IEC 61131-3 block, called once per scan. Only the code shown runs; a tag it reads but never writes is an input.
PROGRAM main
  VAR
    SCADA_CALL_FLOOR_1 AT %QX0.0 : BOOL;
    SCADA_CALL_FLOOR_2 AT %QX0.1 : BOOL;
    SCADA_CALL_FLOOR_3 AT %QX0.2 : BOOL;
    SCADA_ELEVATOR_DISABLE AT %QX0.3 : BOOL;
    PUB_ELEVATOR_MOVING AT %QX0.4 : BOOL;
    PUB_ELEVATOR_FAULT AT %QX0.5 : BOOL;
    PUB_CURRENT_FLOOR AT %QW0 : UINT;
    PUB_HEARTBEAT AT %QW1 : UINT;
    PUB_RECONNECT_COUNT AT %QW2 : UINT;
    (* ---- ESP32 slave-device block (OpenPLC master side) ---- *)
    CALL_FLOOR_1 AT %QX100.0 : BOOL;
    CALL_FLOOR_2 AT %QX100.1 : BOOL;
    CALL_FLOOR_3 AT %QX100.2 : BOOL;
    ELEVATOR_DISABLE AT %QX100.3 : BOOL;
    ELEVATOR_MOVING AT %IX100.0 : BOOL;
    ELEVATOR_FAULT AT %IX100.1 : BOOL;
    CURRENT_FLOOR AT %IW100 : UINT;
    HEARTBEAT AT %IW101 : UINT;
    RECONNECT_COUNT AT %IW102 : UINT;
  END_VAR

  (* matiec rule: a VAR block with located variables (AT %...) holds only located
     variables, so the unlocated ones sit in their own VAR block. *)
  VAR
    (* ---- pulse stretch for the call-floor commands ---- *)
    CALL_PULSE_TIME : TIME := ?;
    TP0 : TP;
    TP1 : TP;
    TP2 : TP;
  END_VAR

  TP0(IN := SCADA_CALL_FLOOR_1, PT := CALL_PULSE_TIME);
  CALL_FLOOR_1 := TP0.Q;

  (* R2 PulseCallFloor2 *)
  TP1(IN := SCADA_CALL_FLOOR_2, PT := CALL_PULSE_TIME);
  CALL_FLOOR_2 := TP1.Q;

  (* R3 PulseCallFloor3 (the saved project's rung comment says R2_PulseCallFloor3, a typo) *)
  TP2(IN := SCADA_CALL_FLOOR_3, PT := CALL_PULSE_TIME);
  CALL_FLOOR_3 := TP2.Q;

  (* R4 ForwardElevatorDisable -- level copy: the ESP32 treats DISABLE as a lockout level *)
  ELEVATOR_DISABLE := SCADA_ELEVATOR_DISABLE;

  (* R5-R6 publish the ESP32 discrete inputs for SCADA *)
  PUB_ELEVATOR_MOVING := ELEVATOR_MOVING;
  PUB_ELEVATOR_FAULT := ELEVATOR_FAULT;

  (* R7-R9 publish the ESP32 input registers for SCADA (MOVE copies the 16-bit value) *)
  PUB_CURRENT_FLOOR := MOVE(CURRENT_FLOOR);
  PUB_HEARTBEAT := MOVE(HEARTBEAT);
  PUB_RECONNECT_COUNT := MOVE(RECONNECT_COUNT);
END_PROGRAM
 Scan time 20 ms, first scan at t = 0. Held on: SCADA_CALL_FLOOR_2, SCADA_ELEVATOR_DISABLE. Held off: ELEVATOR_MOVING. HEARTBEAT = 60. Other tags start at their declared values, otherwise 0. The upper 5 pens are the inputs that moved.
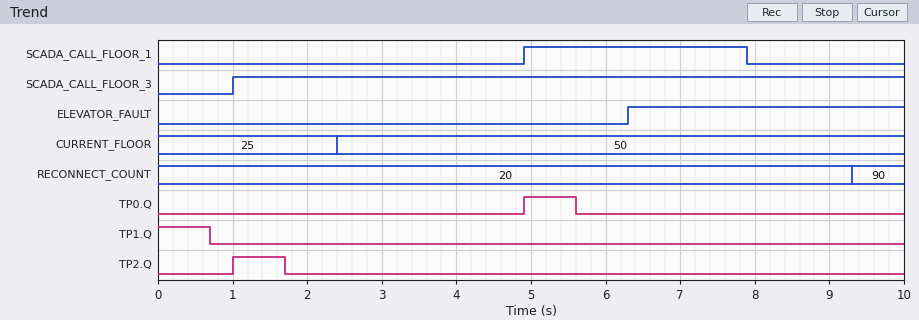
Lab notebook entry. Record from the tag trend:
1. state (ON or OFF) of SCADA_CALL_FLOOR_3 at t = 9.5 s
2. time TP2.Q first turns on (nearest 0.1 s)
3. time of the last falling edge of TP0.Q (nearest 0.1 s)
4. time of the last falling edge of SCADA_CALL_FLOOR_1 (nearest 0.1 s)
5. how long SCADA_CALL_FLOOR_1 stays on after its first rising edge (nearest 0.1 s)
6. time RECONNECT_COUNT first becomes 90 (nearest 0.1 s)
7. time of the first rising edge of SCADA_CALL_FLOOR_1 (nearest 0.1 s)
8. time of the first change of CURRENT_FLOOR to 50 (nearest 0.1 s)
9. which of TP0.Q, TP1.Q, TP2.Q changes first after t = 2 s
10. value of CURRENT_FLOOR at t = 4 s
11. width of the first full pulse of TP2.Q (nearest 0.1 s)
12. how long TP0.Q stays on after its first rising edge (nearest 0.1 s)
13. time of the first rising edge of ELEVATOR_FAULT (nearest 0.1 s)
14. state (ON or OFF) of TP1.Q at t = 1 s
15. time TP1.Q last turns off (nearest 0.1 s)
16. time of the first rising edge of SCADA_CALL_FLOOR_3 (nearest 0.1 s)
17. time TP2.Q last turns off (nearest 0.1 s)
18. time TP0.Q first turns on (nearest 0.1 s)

ON
1.0 s
5.6 s
7.9 s
3.0 s
9.3 s
4.9 s
2.4 s
TP0.Q
50
0.7 s
0.7 s
6.3 s
OFF
0.7 s
1.0 s
1.7 s
4.9 s
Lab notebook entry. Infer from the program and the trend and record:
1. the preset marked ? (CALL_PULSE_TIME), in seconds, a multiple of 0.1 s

0.7 s
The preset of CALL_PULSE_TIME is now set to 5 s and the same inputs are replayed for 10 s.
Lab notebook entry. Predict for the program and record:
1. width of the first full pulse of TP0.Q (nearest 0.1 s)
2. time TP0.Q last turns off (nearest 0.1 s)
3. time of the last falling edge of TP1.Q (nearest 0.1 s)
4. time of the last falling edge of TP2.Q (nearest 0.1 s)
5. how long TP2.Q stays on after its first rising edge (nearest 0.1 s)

5.0 s
9.9 s
5.0 s
6.0 s
5.0 s
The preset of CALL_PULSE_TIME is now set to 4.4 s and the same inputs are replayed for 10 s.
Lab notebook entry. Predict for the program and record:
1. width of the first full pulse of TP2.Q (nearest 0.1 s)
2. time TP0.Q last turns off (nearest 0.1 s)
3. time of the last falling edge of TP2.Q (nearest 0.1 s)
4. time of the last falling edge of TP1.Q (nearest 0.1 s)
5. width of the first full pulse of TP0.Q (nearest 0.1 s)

4.4 s
9.3 s
5.4 s
4.4 s
4.4 s
